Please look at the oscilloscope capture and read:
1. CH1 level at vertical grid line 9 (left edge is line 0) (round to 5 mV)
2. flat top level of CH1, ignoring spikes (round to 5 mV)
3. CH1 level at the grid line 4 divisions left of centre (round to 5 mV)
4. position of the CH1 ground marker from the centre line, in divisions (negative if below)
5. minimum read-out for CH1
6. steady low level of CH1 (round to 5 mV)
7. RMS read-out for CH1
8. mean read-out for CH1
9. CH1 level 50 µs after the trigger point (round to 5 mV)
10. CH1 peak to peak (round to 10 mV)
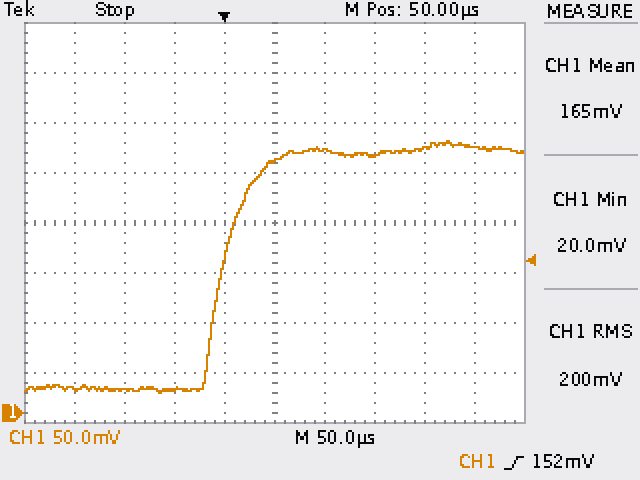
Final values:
265 mV
260 mV
25 mV
-3.8 div
20.0 mV
25 mV
200 mV
165 mV
250 mV
250 mV
